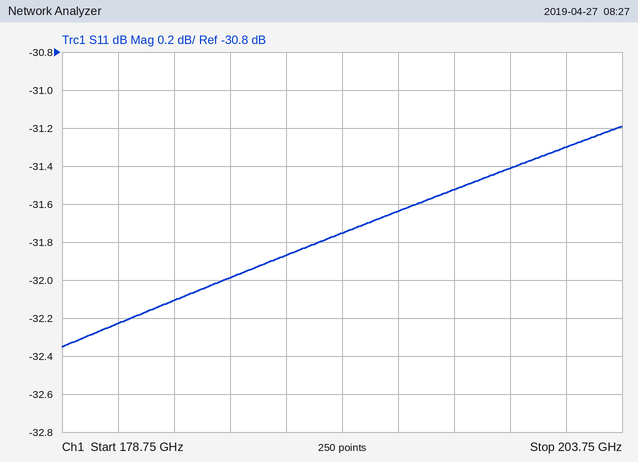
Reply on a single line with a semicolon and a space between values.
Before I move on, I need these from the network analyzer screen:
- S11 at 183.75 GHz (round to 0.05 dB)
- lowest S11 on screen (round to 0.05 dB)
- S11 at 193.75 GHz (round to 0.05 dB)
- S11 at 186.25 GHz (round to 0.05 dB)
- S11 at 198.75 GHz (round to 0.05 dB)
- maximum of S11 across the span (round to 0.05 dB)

-32.10 dB; -32.35 dB; -31.65 dB; -32.00 dB; -31.40 dB; -31.20 dB
